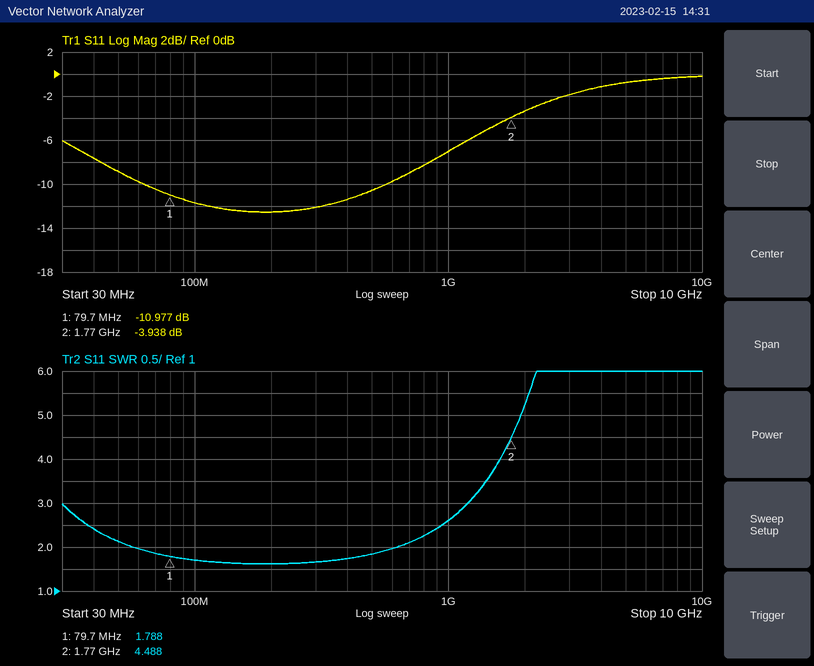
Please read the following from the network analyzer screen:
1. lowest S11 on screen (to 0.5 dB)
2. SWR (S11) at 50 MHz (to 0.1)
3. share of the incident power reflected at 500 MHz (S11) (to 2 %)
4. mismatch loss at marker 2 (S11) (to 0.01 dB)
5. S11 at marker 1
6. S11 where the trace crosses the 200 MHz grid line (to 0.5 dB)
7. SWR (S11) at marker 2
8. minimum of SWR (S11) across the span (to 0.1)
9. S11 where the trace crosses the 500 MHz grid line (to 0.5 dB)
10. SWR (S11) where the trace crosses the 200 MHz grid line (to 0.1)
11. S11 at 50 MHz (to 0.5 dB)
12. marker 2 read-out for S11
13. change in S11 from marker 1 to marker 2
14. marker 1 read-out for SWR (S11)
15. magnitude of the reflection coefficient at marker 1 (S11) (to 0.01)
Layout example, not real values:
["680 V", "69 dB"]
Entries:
["-12.5 dB", "2.1", "8 %", "2.25 dB", "-10.977 dB", "-12.5 dB", "4.488", "1.6", "-10.5 dB", "1.6", "-9.0 dB", "-3.938 dB", "7.039 dB", "1.788", "0.28"]
